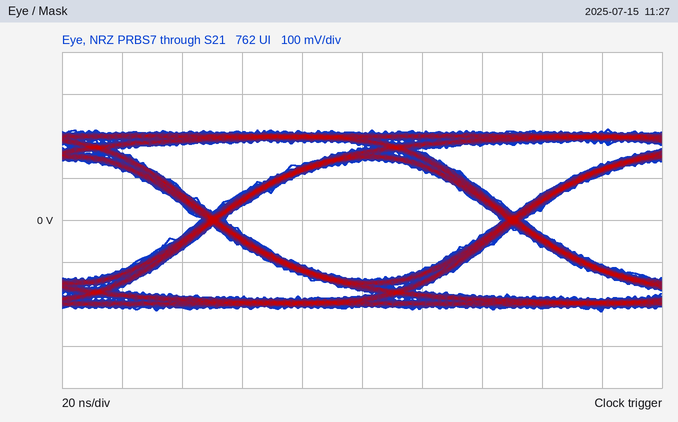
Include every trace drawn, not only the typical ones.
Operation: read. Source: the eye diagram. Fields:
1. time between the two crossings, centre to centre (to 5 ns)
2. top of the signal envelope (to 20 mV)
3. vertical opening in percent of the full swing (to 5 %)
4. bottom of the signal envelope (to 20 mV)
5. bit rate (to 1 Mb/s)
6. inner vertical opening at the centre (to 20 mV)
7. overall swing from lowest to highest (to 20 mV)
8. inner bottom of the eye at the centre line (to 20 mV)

100 ns
220 mV
65 %
-220 mV
10 Mb/s
280 mV
440 mV
-140 mV
